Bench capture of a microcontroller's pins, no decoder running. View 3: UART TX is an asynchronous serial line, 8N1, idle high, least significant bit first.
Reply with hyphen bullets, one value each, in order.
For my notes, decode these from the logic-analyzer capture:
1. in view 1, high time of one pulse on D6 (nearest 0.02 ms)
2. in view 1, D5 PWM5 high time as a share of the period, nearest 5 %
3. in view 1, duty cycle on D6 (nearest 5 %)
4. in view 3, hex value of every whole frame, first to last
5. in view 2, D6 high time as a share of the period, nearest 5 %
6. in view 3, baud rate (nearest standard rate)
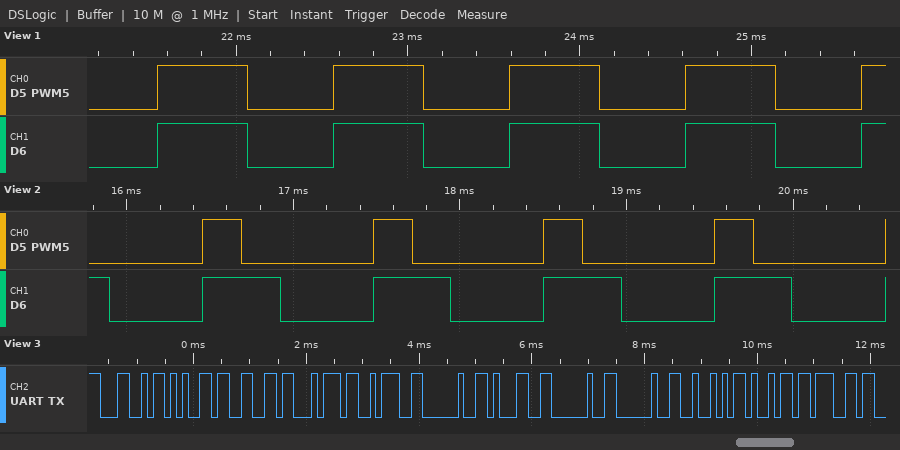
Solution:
- 0.52 ms
- 50 %
- 50 %
- 4C 65 66 74 3A 20 31 20 20 52 69 67
- 45 %
- 9600 baud
